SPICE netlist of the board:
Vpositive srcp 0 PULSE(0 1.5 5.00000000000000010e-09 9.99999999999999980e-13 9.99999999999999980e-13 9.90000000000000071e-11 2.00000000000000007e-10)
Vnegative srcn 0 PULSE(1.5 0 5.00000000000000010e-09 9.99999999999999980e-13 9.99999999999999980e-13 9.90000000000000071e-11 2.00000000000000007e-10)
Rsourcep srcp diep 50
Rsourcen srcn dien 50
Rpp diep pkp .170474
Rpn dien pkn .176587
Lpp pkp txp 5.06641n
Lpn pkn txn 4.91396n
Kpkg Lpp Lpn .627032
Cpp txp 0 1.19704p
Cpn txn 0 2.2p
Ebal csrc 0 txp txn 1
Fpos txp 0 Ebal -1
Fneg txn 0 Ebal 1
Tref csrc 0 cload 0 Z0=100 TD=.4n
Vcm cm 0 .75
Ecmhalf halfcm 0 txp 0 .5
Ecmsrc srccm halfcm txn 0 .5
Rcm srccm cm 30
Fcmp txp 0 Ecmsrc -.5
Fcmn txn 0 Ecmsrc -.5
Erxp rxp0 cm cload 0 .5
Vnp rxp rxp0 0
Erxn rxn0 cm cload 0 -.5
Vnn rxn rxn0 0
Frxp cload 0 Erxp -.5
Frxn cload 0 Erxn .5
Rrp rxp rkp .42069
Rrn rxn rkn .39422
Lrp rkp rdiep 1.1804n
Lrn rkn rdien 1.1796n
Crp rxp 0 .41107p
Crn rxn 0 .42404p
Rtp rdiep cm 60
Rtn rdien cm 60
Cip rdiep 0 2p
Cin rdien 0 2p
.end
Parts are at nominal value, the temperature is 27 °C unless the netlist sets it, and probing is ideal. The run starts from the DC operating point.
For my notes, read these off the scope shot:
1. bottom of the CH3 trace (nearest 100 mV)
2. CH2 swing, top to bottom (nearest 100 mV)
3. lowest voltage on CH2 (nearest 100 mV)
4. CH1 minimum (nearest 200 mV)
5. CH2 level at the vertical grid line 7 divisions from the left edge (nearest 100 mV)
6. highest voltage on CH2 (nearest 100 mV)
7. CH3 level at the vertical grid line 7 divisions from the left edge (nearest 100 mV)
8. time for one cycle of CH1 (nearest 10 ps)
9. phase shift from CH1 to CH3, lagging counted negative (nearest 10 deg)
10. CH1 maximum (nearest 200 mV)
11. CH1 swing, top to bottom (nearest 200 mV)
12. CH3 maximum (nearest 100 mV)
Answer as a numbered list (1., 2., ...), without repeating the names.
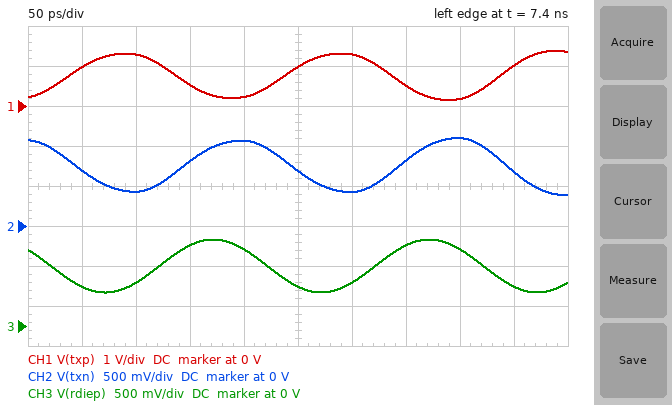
1. 400 mV
2. 700 mV
3. 400 mV
4. 200 mV
5. 800 mV
6. 1.1 V
7. 1.0 V
8. 200 ps
9. -150 deg
10. 1.4 V
11. 1.2 V
12. 1.1 V
